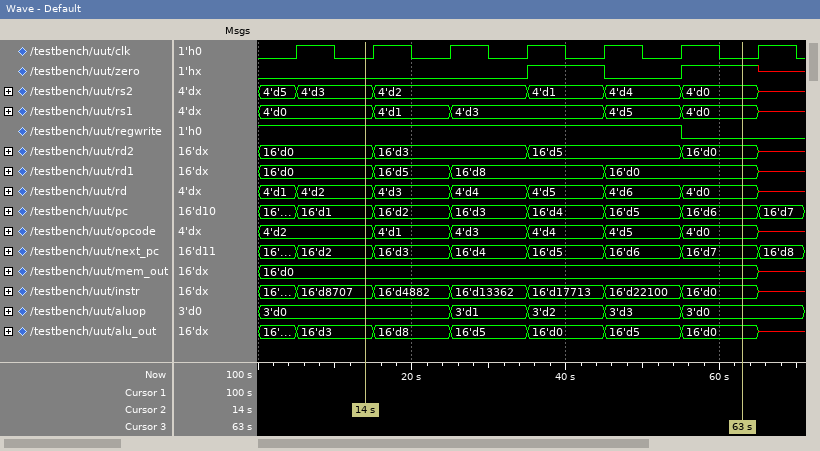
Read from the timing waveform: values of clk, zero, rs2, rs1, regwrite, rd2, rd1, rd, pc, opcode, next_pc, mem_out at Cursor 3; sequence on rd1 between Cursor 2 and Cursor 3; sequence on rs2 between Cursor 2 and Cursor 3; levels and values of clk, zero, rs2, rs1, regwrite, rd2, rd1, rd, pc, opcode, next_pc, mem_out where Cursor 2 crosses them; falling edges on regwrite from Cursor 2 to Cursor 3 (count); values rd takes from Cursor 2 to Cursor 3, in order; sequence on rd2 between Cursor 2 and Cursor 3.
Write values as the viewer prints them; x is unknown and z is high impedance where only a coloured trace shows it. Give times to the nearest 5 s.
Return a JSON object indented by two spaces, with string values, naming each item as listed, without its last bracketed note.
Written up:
{
  "values of clk, zero, rs2, rs1, regwrite, rd2, rd1, rd, pc, opcode, next_pc, mem_out at Cursor 3": "clk=0, zero=1, rs2=4'd0, rs1=4'd0, regwrite=0, rd2=16'd0, rd1=16'd0, rd=4'd0, pc=16'd6, opcode=4'd0, next_pc=16'd7, mem_out=16'd0",
  "sequence on rd1 between Cursor 2 and Cursor 3": "16'd0, 16'd5, 16'd8, 16'd0",
  "sequence on rs2 between Cursor 2 and Cursor 3": "4'd3, 4'd2, 4'd1, 4'd4, 4'd0",
  "levels and values of clk, zero, rs2, rs1, regwrite, rd2, rd1, rd, pc, opcode, next_pc, mem_out where Cursor 2 crosses them": "clk=0, zero=0, rs2=4'd3, rs1=4'd0, regwrite=1, rd2=16'd0, rd1=16'd0, rd=4'd2, pc=16'd1, opcode=4'd2, next_pc=16'd2, mem_out=16'd0",
  "falling edges on regwrite from Cursor 2 to Cursor 3": "1",
  "values rd takes from Cursor 2 to Cursor 3, in order": "4'd2, 4'd3, 4'd4, 4'd5, 4'd6, 4'd0",
  "sequence on rd2 between Cursor 2 and Cursor 3": "16'd0, 16'd3, 16'd5, 16'd0"
}
